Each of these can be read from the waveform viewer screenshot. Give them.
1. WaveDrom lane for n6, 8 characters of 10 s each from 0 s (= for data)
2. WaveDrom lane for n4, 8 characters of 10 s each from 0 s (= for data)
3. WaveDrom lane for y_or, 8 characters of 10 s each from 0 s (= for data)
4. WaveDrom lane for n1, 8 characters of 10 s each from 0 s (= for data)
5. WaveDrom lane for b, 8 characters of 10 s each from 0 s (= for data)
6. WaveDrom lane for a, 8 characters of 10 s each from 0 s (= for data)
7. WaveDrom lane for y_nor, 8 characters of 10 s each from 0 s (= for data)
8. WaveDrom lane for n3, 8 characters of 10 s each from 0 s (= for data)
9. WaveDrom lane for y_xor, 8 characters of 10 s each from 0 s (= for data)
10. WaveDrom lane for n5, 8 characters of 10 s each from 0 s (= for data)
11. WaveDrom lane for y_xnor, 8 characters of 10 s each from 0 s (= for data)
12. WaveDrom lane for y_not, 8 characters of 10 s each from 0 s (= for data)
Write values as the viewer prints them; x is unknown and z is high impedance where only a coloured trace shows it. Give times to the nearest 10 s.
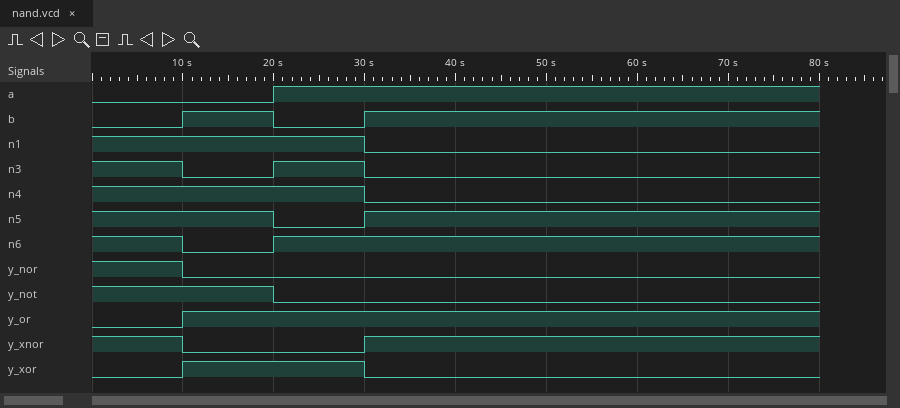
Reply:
{name: 'n6', wave: '101.....'}
{name: 'n4', wave: '1..0....'}
{name: 'y_or', wave: '01......'}
{name: 'n1', wave: '1..0....'}
{name: 'b', wave: '0101....'}
{name: 'a', wave: '0.1.....'}
{name: 'y_nor', wave: '10......'}
{name: 'n3', wave: '1010....'}
{name: 'y_xor', wave: '01.0....'}
{name: 'n5', wave: '1.01....'}
{name: 'y_xnor', wave: '10.1....'}
{name: 'y_not', wave: '1.0.....'}
